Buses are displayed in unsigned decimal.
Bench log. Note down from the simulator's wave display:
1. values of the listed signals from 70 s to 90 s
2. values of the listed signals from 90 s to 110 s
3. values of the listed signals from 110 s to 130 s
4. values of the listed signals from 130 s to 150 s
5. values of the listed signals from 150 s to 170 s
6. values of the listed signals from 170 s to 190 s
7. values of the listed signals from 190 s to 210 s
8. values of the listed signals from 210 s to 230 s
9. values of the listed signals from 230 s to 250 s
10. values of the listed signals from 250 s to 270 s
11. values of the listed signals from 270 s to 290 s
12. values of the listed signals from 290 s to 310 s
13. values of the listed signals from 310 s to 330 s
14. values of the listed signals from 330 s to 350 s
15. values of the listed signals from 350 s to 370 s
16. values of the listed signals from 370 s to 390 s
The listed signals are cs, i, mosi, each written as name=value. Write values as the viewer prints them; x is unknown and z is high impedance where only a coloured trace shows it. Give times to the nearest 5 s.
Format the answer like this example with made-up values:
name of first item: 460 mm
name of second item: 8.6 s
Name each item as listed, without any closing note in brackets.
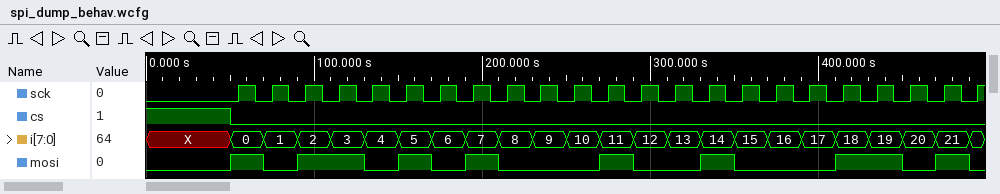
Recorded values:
values of the listed signals from 70 s to 90 s: cs=0, i=1, mosi=0
values of the listed signals from 90 s to 110 s: cs=0, i=2, mosi=1
values of the listed signals from 110 s to 130 s: cs=0, i=3, mosi=1
values of the listed signals from 130 s to 150 s: cs=0, i=4, mosi=0
values of the listed signals from 150 s to 170 s: cs=0, i=5, mosi=1
values of the listed signals from 170 s to 190 s: cs=0, i=6, mosi=0
values of the listed signals from 190 s to 210 s: cs=0, i=7, mosi=1
values of the listed signals from 210 s to 230 s: cs=0, i=8, mosi=0
values of the listed signals from 230 s to 250 s: cs=0, i=9, mosi=0
values of the listed signals from 250 s to 270 s: cs=0, i=10, mosi=0
values of the listed signals from 270 s to 290 s: cs=0, i=11, mosi=1
values of the listed signals from 290 s to 310 s: cs=0, i=12, mosi=0
values of the listed signals from 310 s to 330 s: cs=0, i=13, mosi=0
values of the listed signals from 330 s to 350 s: cs=0, i=14, mosi=1
values of the listed signals from 350 s to 370 s: cs=0, i=15, mosi=0
values of the listed signals from 370 s to 390 s: cs=0, i=16, mosi=0
